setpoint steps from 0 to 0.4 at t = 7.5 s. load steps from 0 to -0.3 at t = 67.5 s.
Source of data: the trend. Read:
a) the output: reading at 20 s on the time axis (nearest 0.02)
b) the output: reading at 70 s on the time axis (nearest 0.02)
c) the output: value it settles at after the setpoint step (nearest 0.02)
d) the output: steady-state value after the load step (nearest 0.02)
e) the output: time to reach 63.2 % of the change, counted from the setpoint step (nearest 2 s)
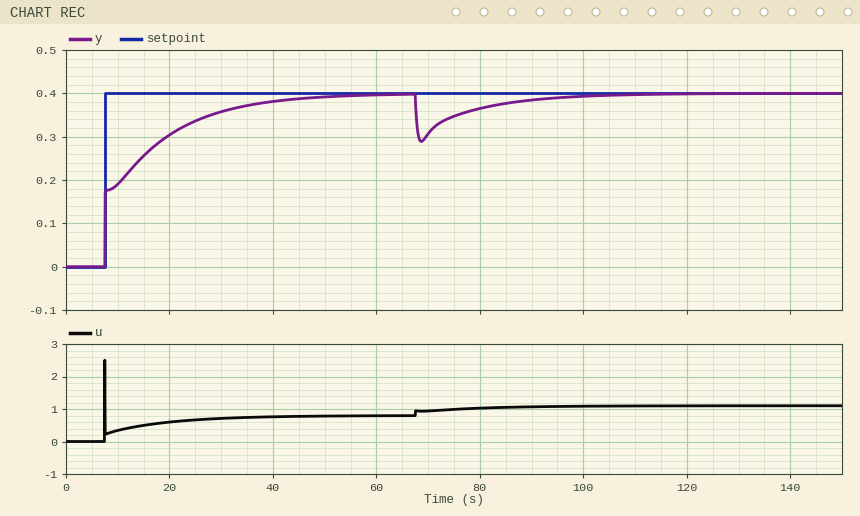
0.30
0.30
0.40
0.40
8 s
